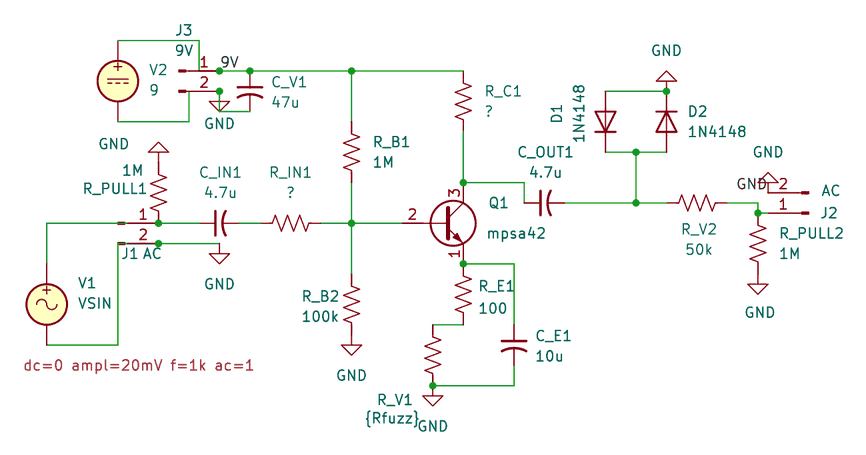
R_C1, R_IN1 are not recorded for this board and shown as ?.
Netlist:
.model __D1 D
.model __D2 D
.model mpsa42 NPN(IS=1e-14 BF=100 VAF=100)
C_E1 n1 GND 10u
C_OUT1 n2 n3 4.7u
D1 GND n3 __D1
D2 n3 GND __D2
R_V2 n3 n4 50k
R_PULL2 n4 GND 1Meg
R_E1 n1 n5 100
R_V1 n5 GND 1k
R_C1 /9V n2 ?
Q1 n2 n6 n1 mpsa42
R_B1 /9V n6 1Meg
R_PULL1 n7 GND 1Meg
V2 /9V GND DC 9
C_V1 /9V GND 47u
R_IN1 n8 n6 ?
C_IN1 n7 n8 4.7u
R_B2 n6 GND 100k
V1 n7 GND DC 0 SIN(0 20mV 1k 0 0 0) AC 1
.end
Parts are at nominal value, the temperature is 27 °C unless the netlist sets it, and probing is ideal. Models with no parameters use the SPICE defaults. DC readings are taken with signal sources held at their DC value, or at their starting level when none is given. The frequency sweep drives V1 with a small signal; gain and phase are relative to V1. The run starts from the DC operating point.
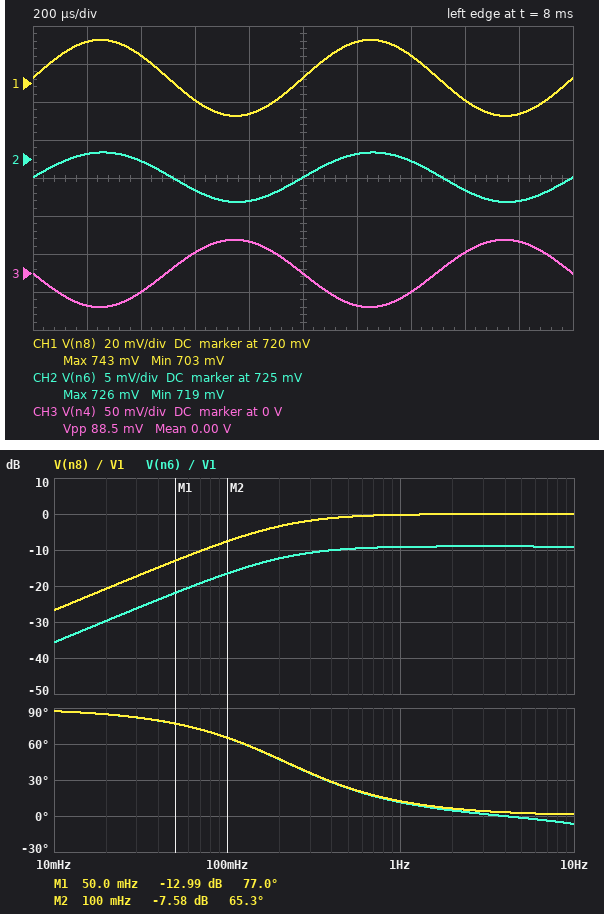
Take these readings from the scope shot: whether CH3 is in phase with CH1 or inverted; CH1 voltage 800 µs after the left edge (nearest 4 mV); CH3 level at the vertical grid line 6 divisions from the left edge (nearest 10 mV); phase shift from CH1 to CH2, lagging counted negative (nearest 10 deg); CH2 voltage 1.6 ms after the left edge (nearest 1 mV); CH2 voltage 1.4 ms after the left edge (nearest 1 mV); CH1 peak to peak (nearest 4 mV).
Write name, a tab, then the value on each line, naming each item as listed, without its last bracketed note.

whether CH3 is in phase with CH1 or inverted	inverted
CH1 voltage 800 µs after the left edge	704 mV
CH3 level at the vertical grid line 6 divisions from the left edge	-40 mV
phase shift from CH1 to CH2, lagging counted negative	0 deg
CH2 voltage 1.6 ms after the left edge	721 mV
CH2 voltage 1.4 ms after the left edge	725 mV
CH1 peak to peak	40 mV
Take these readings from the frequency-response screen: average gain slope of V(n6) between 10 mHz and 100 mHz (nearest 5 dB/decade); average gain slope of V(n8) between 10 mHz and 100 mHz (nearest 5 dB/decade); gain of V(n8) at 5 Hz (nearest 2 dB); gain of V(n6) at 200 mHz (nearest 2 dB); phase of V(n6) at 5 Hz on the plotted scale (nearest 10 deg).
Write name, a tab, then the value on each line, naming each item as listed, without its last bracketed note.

average gain slope of V(n6) between 10 mHz and 100 mHz	20 dB/decade
average gain slope of V(n8) between 10 mHz and 100 mHz	20 dB/decade
gain of V(n8) at 5 Hz	0 dB
gain of V(n6) at 200 mHz	-12 dB
phase of V(n6) at 5 Hz on the plotted scale	0 deg
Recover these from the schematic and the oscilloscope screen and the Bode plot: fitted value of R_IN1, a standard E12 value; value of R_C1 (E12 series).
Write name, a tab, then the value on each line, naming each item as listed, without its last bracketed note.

fitted value of R_IN1, a standard E12 value	100 kΩ
value of R_C1	3.3 kΩ
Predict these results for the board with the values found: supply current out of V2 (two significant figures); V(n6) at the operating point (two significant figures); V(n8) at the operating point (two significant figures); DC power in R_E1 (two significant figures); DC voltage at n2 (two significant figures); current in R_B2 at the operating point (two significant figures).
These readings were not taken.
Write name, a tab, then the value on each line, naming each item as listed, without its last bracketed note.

supply current out of V2	120 µA
V(n6) at the operating point	720 mV
V(n8) at the operating point	720 mV
DC power in R_E1	1.3 µW
DC voltage at n2	8.6 V
current in R_B2 at the operating point	7.2 µA
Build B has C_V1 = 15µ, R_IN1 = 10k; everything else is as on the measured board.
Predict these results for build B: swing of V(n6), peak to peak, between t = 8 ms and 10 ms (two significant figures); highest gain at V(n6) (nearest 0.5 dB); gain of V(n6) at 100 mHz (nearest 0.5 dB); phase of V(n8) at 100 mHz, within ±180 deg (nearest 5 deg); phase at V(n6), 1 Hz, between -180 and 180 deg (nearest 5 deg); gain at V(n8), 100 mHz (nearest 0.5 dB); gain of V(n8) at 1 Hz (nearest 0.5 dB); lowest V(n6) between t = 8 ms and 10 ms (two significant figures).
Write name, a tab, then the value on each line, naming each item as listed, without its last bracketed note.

swing of V(n6), peak to peak, between t = 8 ms and 10 ms	27 mV
highest gain at V(n6)	-1.5 dB
gain of V(n6) at 100 mHz	-16.0 dB
phase of V(n8) at 100 mHz, within ±180 deg	80 deg
phase at V(n6), 1 Hz, between -180 and 180 deg	25 deg
gain at V(n8), 100 mHz	-14.5 dB
gain of V(n8) at 1 Hz	-1.0 dB
lowest V(n6) between t = 8 ms and 10 ms	710 mV
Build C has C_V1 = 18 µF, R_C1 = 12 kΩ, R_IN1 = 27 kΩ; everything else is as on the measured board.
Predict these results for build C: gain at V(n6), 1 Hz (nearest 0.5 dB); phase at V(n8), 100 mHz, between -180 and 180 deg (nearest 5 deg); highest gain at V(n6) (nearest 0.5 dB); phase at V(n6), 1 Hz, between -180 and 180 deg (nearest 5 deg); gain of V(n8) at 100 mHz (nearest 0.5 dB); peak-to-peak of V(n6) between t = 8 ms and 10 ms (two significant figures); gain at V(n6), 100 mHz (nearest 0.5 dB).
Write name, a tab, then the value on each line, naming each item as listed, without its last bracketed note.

gain at V(n6), 1 Hz	-4.0 dB
phase at V(n8), 100 mHz, between -180 and 180 deg	75 deg
highest gain at V(n6)	-3.5 dB
phase at V(n6), 1 Hz, between -180 and 180 deg	20 deg
gain of V(n8) at 100 mHz	-12.5 dB
peak-to-peak of V(n6) between t = 8 ms and 10 ms	17 mV
gain at V(n6), 100 mHz	-16.0 dB
